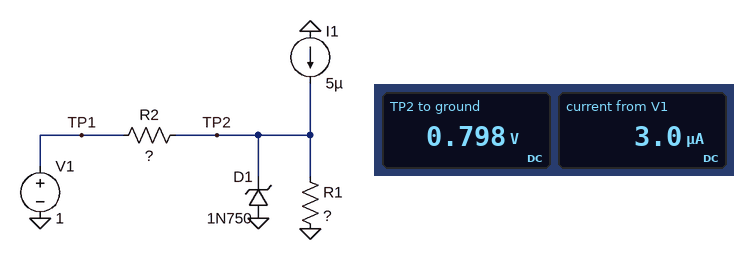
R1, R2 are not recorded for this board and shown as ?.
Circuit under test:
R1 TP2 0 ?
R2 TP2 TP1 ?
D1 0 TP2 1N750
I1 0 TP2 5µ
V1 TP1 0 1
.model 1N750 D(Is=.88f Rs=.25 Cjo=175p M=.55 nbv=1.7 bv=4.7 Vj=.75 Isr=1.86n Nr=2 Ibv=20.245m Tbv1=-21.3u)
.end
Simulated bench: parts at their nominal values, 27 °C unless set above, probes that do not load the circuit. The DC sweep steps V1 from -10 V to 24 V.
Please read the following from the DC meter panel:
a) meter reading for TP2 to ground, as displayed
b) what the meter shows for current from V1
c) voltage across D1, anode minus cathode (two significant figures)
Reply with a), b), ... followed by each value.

a) 0.798 V
b) 3.0 µA
c) -800 mV
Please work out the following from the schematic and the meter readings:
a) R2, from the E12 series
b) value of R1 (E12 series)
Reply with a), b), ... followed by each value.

a) 68 kΩ
b) 100 kΩ
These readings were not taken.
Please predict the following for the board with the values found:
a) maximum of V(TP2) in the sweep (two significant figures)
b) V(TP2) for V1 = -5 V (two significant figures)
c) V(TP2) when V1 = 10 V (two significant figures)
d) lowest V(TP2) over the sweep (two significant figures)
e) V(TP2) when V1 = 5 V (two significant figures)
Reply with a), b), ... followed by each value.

a) 4.5 V
b) -570 mV
c) 4.4 V
d) -610 mV
e) 3.2 V
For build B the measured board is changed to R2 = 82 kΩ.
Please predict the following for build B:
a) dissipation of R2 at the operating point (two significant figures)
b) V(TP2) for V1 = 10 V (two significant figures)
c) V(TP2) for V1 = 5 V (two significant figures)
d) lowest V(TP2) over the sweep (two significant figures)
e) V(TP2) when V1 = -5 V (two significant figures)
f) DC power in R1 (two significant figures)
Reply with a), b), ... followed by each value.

a) 620 nW
b) 4.4 V
c) 3.0 V
d) -600 mV
e) -560 mV
f) 6.0 µW
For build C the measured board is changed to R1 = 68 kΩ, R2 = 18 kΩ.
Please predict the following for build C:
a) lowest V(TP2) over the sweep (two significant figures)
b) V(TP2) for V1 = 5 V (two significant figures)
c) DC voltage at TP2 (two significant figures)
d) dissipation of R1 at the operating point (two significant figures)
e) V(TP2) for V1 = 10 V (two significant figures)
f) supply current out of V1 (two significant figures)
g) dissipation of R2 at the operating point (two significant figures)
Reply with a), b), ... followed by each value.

a) -680 mV
b) 4.0 V
c) 860 mV
d) 11 µW
e) 4.5 V
f) 7.7 µA
g) 1.1 µW
